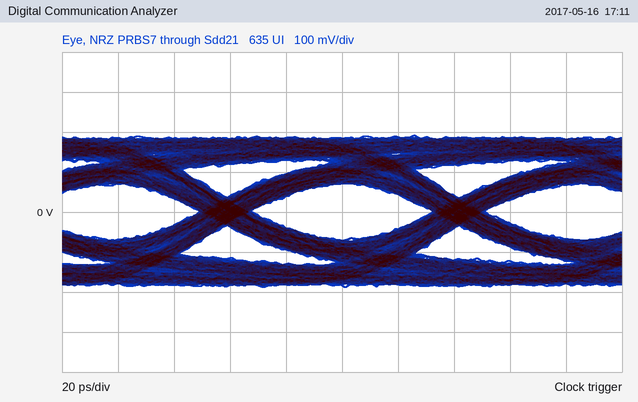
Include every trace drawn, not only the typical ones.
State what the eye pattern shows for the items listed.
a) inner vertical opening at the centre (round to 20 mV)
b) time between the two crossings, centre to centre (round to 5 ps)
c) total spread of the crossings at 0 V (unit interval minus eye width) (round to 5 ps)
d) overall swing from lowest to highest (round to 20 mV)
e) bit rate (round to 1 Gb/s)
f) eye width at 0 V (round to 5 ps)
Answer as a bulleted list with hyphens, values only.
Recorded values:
- 140 mV
- 85 ps
- 20 ps
- 380 mV
- 12 Gb/s
- 65 ps
